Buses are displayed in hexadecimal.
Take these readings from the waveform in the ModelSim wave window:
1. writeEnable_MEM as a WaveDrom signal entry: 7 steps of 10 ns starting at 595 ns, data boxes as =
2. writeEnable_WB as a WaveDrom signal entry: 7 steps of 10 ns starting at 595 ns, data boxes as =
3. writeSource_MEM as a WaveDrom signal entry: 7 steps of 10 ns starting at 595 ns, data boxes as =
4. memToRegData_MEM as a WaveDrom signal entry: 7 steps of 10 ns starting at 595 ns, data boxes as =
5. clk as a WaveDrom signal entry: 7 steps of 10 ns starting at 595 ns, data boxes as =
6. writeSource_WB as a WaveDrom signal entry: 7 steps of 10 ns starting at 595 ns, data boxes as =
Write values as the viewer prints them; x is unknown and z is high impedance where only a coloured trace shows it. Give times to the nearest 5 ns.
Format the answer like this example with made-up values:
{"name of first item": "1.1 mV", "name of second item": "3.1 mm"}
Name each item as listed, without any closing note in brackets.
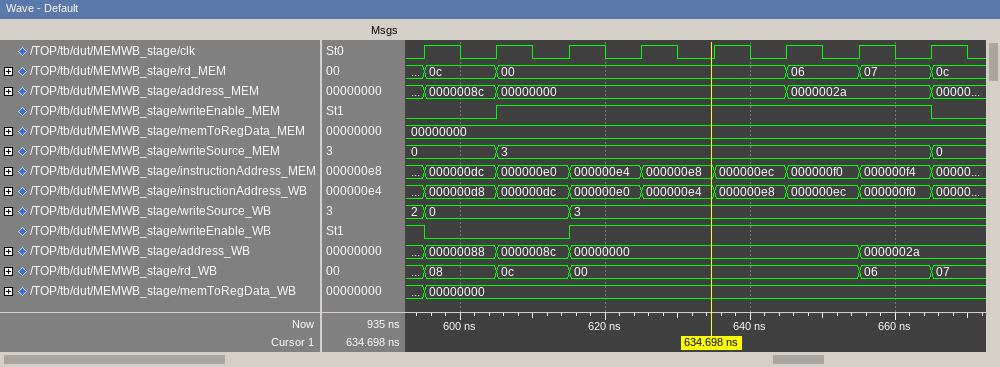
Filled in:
{"writeEnable_MEM as a WaveDrom signal entry: 7 steps of 10 ns starting at 595 ns, data boxes as =": "{name: 'writeEnable_MEM', wave: '01.....'}", "writeEnable_WB as a WaveDrom signal entry: 7 steps of 10 ns starting at 595 ns, data boxes as =": "{name: 'writeEnable_WB', wave: '0.1....'}", "writeSource_MEM as a WaveDrom signal entry: 7 steps of 10 ns starting at 595 ns, data boxes as =": "{name: 'writeSource_MEM', wave: '==.....', data: '0 3'}", "memToRegData_MEM as a WaveDrom signal entry: 7 steps of 10 ns starting at 595 ns, data boxes as =": "{name: 'memToRegData_MEM', wave: '=......', data: '00000000'}", "clk as a WaveDrom signal entry: 7 steps of 10 ns starting at 595 ns, data boxes as =": "{name: 'clk', wave: 'p......'}", "writeSource_WB as a WaveDrom signal entry: 7 steps of 10 ns starting at 595 ns, data boxes as =": "{name: 'writeSource_WB', wave: '=.=....', data: '0 3'}"}
